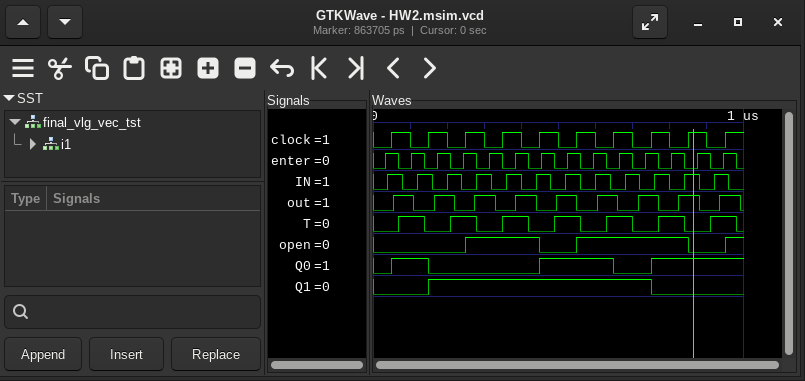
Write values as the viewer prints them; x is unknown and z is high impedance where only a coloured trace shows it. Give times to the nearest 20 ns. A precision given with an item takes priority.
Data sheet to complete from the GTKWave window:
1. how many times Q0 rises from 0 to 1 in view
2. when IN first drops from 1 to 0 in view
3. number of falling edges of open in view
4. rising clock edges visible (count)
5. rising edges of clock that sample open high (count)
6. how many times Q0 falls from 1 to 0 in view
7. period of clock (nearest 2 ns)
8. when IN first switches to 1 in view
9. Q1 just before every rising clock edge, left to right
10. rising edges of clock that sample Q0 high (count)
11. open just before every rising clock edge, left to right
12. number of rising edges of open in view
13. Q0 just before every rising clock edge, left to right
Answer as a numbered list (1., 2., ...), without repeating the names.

1. 3
2. 80 ns
3. 2
4. 10
5. 5
6. 2
7. 100 ns
8. 40 ns
9. 0 0 1 1 1 1 1 1 0 0
10. 5
11. 0 0 0 1 1 0 1 1 1 0
12. 3
13. 0 1 0 0 0 1 1 0 1 1
